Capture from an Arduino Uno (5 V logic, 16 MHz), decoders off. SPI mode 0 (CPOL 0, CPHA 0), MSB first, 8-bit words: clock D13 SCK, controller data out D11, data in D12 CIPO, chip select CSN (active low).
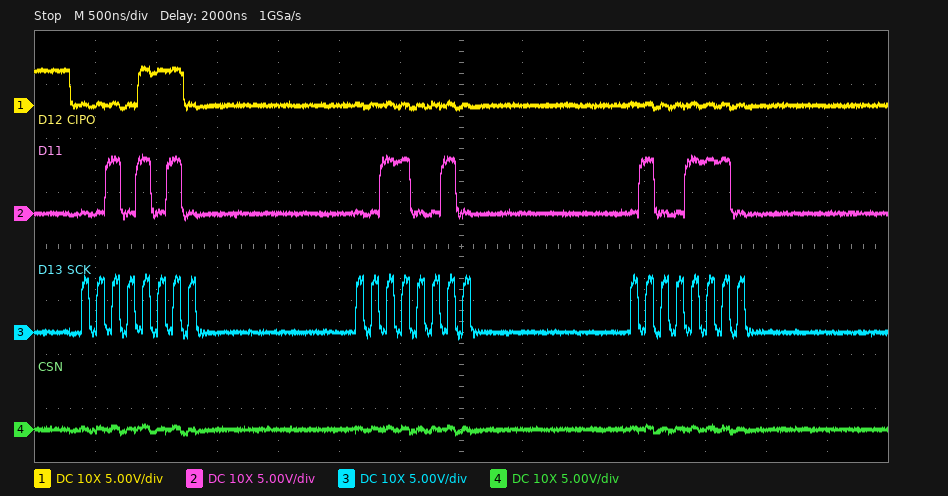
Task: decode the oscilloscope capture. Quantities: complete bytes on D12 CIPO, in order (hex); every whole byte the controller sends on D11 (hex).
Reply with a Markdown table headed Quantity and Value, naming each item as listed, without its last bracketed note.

| Quantity | Value |
|---|---|
| complete bytes on D12 CIPO, in order | 0x0E 0x00 0x00 |
| every whole byte the controller sends on D11 | 0x2A 0x32 0x4E |
